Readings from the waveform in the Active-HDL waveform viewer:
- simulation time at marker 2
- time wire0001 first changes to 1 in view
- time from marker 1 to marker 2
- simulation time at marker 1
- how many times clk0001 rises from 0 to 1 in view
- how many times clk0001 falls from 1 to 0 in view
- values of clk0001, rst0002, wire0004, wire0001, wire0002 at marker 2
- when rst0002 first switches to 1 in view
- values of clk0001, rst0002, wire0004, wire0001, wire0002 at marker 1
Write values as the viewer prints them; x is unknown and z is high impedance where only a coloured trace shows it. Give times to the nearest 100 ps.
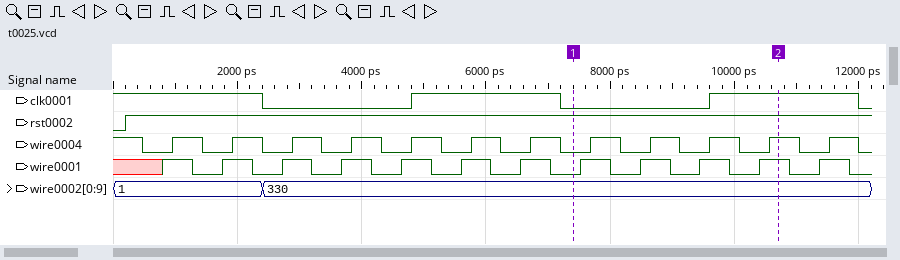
10700 ps
800 ps
3300 ps
7400 ps
2
3
clk0001=1, rst0002=1, wire0004=1, wire0001=1, wire0002=330
200 ps
clk0001=0, rst0002=1, wire0004=0, wire0001=0, wire0002=330
